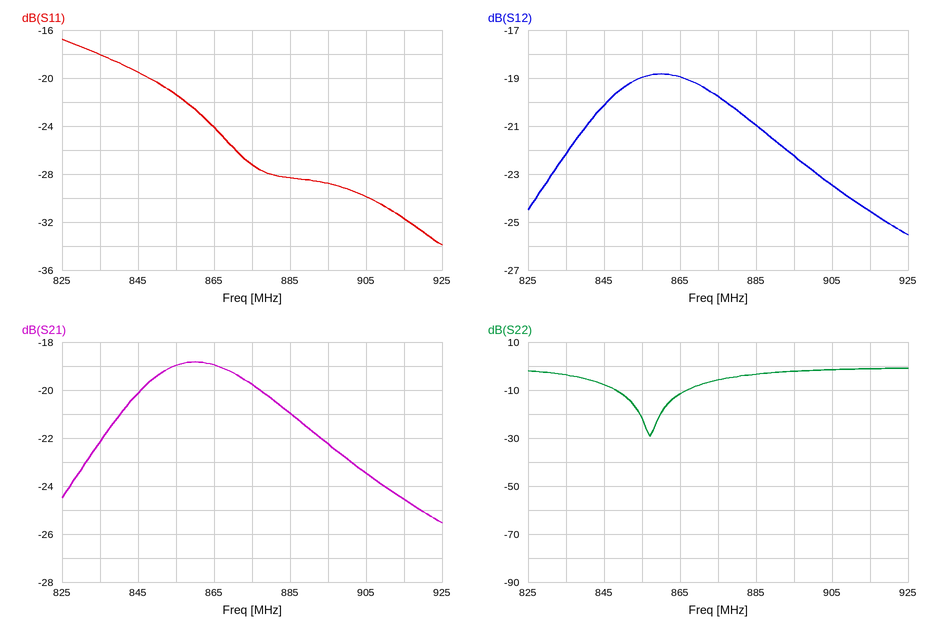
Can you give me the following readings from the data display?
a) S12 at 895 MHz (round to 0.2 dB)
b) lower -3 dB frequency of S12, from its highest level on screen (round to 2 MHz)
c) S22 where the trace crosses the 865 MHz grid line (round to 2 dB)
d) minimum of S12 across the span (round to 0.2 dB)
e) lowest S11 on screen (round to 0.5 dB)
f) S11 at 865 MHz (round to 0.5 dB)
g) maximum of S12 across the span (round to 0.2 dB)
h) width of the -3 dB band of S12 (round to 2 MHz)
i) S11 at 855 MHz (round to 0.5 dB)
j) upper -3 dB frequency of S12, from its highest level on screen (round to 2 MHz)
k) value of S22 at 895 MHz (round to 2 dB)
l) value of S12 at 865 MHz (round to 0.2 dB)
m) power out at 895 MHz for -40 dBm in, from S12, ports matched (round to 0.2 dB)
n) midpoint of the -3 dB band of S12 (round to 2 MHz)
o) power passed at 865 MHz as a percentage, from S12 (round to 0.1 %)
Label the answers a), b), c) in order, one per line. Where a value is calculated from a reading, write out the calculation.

a) -22.2 dB
b) 836 MHz
c) -12 dB
d) -25.6 dB
e) -34.0 dB
f) -24.0 dB
g) -18.8 dB
h) 892 MHz − 836 MHz = 56 MHz
i) -21.5 dB
j) 892 MHz
k) -2 dB
l) -19.0 dB
m) -40 dBm + (-22.2 dB) = -62.2 dBm
n) 864 MHz
o) 10^(-19/10) ≈ 1.3 %
